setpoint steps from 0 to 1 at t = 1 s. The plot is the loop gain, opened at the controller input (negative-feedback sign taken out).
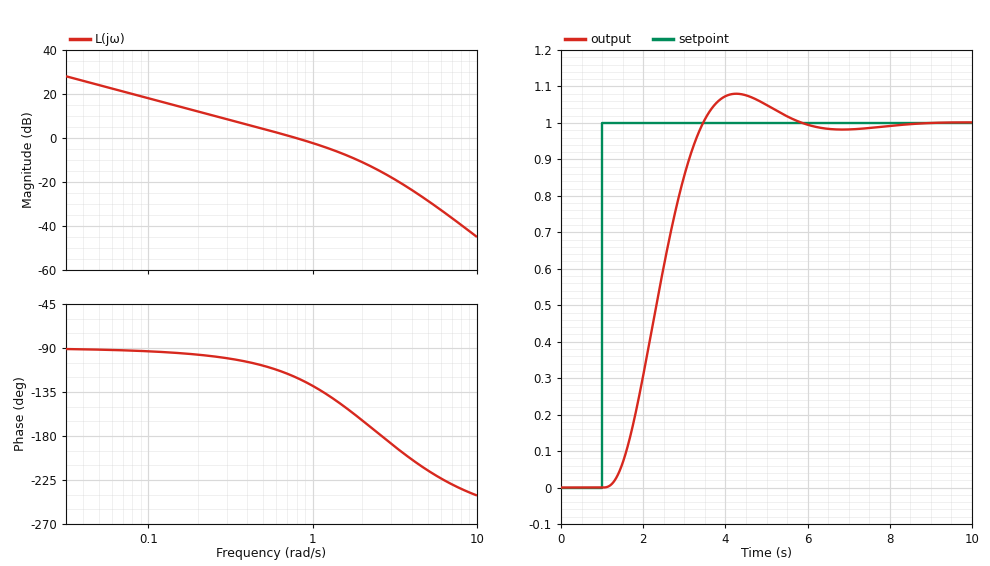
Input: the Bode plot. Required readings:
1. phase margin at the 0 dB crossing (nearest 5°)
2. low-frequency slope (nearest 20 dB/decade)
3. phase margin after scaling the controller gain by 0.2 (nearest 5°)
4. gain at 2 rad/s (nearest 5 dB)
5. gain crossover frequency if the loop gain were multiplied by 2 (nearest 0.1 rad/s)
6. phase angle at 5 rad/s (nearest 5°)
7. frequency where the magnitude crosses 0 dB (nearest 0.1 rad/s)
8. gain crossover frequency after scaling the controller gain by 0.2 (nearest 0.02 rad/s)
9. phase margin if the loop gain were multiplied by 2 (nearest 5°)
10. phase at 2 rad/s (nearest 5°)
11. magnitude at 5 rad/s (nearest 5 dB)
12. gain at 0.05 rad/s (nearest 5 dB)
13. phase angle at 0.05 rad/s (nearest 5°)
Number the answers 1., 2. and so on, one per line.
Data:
1. 60°
2. -20 dB/decade
3. 85°
4. -10 dB
5. 1.4 rad/s
6. -215°
7. 0.8 rad/s
8. 0.16 rad/s
9. 35°
10. -165°
11. -30 dB
12. 25 dB
13. -90°
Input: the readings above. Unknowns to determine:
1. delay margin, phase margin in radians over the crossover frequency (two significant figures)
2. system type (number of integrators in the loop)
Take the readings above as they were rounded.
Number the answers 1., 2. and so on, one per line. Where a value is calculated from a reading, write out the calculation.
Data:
1. 60 × π / 180 / 0.8 = 1.3 s
2. 1
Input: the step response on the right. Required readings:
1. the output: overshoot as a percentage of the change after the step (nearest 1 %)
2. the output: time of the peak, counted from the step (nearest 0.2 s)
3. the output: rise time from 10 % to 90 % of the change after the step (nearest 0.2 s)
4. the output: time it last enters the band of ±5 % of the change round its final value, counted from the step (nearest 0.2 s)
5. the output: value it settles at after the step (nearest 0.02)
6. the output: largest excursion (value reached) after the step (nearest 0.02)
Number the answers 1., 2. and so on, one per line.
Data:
1. 8 %
2. 3.2 s
3. 1.6 s
4. 4.0 s
5. 1.00
6. 1.08
